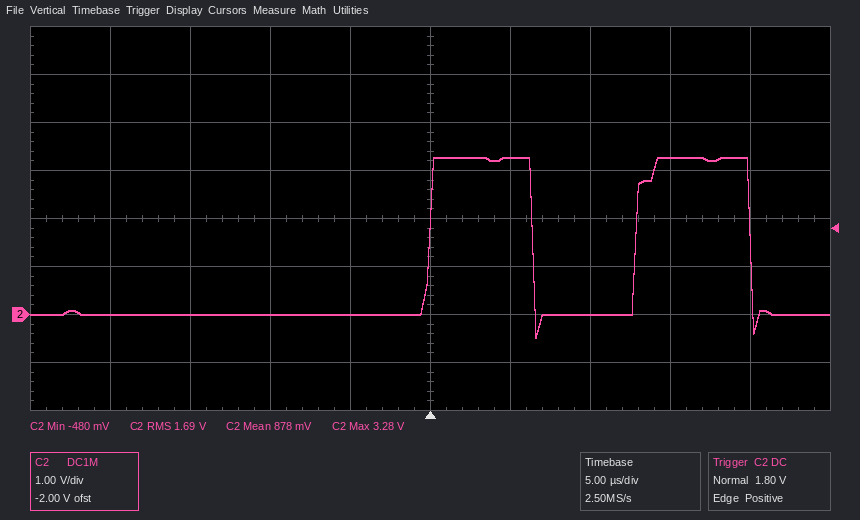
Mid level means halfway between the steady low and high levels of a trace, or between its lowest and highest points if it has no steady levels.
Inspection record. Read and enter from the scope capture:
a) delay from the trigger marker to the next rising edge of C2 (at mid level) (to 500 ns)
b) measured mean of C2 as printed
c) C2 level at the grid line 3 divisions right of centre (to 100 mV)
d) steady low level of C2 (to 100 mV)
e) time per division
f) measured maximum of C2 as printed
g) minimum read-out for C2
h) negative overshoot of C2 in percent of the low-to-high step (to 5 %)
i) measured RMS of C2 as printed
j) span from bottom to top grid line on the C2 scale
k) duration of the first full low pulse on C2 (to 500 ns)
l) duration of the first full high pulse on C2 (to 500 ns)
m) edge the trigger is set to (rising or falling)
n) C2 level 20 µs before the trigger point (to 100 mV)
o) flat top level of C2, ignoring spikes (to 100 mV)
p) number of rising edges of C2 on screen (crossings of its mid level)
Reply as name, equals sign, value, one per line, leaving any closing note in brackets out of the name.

delay from the trigger marker to the next rising edge of C2 (at mid level) = 13.0 µs
measured mean of C2 as printed = 878 mV
C2 level at the grid line 3 divisions right of centre = 3.3 V
steady low level of C2 = 0.0 V
time per division = 5 µs
measured maximum of C2 as printed = 3.28 V
minimum read-out for C2 = -480 mV
negative overshoot of C2 in percent of the low-to-high step = 15 %
measured RMS of C2 as printed = 1.69 V
span from bottom to top grid line on the C2 scale = 8 V
duration of the first full low pulse on C2 = 6.5 µs
duration of the first full high pulse on C2 = 6.5 µs
edge the trigger is set to = rising
C2 level 20 µs before the trigger point = 0.0 V
flat top level of C2, ignoring spikes = 3.3 V
number of rising edges of C2 on screen = 2
